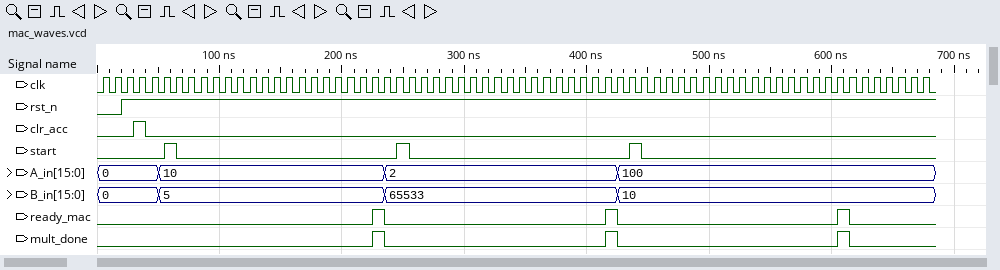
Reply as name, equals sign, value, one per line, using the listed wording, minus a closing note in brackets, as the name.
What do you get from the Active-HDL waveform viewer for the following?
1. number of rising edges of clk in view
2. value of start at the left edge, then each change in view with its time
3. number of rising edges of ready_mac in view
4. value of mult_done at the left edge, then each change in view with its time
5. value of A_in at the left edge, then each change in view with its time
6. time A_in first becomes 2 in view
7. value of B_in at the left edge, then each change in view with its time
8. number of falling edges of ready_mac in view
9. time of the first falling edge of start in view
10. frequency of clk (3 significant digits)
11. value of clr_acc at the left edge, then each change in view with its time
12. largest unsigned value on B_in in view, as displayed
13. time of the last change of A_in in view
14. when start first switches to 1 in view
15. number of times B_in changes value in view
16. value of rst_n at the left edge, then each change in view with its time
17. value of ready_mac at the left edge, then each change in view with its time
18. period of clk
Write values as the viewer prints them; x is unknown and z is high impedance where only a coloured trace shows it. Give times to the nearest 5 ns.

number of rising edges of clk in view = 68
value of start at the left edge, then each change in view with its time = 0, 1 at 55 ns, 0 at 65 ns, 1 at 245 ns, 0 at 255 ns, 1 at 435 ns, 0 at 445 ns
number of rising edges of ready_mac in view = 3
value of mult_done at the left edge, then each change in view with its time = 0, 1 at 225 ns, 0 at 235 ns, 1 at 415 ns, 0 at 425 ns, 1 at 605 ns, 0 at 615 ns
value of A_in at the left edge, then each change in view with its time = 0, 10 at 50 ns, 2 at 235 ns, 100 at 425 ns
time A_in first becomes 2 in view = 235 ns
value of B_in at the left edge, then each change in view with its time = 0, 5 at 50 ns, 65533 at 235 ns, 10 at 425 ns
number of falling edges of ready_mac in view = 3
time of the first falling edge of start in view = 65 ns
frequency of clk = 100 MHz
value of clr_acc at the left edge, then each change in view with its time = 0, 1 at 30 ns, 0 at 40 ns
largest unsigned value on B_in in view, as displayed = 65533
time of the last change of A_in in view = 425 ns
when start first switches to 1 in view = 55 ns
number of times B_in changes value in view = 3
value of rst_n at the left edge, then each change in view with its time = 0, 1 at 20 ns
value of ready_mac at the left edge, then each change in view with its time = 0, 1 at 225 ns, 0 at 235 ns, 1 at 415 ns, 0 at 425 ns, 1 at 605 ns, 0 at 615 ns
period of clk = 10 ns
